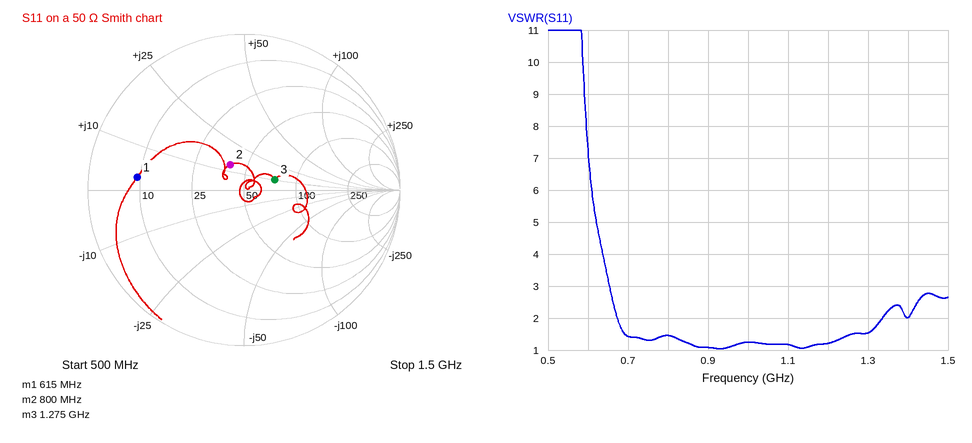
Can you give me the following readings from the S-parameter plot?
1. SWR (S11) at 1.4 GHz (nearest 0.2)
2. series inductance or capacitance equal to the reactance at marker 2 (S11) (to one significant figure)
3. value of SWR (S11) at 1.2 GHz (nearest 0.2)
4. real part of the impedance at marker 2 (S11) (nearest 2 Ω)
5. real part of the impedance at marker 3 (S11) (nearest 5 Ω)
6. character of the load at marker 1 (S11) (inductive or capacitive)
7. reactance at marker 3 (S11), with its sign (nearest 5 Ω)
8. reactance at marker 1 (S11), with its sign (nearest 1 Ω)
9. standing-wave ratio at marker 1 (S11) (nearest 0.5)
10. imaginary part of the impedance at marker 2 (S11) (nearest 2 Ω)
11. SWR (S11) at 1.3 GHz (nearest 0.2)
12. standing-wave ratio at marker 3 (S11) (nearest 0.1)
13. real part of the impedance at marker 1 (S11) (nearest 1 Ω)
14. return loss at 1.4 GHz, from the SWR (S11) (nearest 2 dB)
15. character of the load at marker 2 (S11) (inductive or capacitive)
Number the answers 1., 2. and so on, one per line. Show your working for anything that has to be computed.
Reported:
1. 2.0
2. L = 14 Ω/(2π × 800 MHz) ≈ 3 nH
3. 1.2
4. 40 Ω
5. 75 Ω
6. inductive
7. +10 Ω
8. +3 Ω
9. 5.5
10. +14 Ω
11. 1.6
12. 1.5
13. 9 Ω
14. −20 log10((2 − 1)/(2 + 1)) ≈ 10 dB
15. inductive
